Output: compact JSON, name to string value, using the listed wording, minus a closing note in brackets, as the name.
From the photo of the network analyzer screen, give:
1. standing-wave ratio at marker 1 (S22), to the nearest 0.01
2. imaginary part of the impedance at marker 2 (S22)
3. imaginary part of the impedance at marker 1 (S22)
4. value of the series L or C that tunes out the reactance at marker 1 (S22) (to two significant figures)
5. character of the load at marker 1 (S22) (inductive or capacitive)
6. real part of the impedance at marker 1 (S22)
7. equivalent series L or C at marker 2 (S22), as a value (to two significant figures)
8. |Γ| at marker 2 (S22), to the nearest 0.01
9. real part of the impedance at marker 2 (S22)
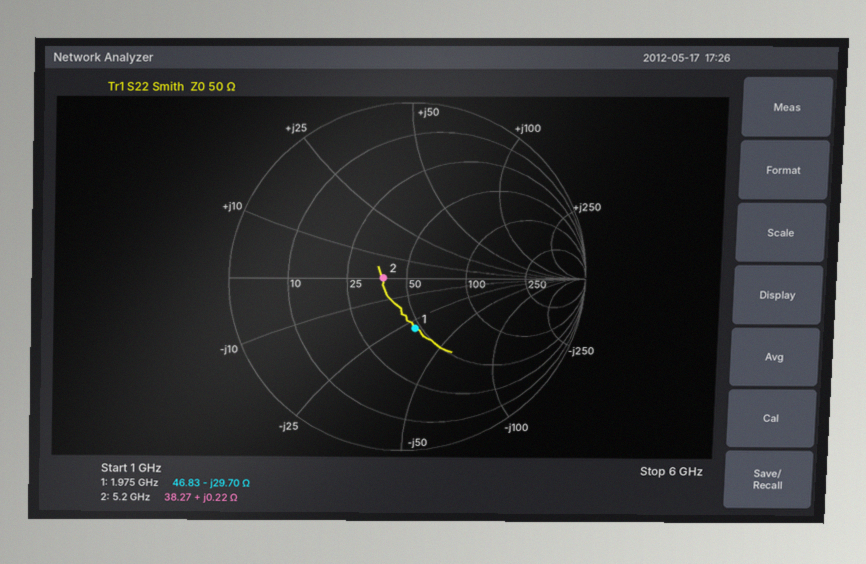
{"standing-wave ratio at marker 1 (S22), to the nearest 0.01": "1.84", "imaginary part of the impedance at marker 2": "+0.22 Ω", "imaginary part of the impedance at marker 1": "-29.70 Ω", "value of the series L or C that tunes out the reactance at marker 1 (S22)": "2.4 nH", "character of the load at marker 1 (S22)": "capacitive", "real part of the impedance at marker 1": "46.83 Ω", "equivalent series L or C at marker 2 (S22), as a value": "6.7 pH", "|Γ| at marker 2 (S22), to the nearest 0.01": "0.13", "real part of the impedance at marker 2": "38.27 Ω"}
